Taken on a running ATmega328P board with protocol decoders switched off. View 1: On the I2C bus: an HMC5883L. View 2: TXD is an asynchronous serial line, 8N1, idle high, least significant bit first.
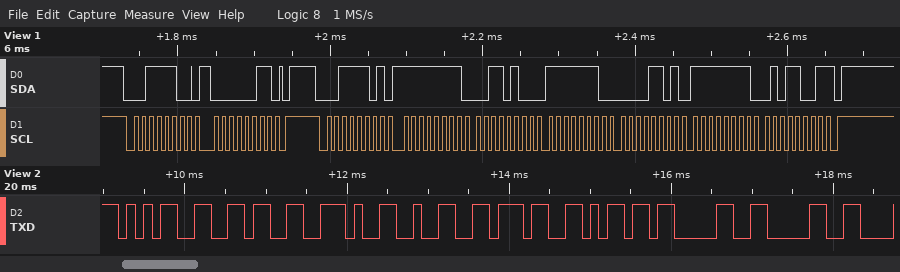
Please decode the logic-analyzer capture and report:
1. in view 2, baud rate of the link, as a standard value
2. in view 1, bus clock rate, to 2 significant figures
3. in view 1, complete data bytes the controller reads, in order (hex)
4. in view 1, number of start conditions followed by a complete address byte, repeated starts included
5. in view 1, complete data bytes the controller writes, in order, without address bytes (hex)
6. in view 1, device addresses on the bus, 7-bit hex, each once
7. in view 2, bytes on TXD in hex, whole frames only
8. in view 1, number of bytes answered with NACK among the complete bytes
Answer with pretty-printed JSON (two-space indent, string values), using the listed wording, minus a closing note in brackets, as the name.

{
  "in view 2, baud rate of the link, as a standard value": "9600 baud",
  "in view 1, bus clock rate, to 2 significant figures": "100 kHz",
  "in view 1, complete data bytes the controller reads, in order": "FF 34 FE 0D FF 59",
  "in view 1, number of start conditions followed by a complete address byte, repeated starts included": "2",
  "in view 1, complete data bytes the controller writes, in order, without address bytes": "03",
  "in view 1, device addresses on the bus, 7-bit hex, each once": "0x1E",
  "in view 2, bytes on TXD in hex, whole frames only": "35 36 2E 32 37 6D 30 30",
  "in view 1, number of bytes answered with NACK among the complete bytes": "1"
}
